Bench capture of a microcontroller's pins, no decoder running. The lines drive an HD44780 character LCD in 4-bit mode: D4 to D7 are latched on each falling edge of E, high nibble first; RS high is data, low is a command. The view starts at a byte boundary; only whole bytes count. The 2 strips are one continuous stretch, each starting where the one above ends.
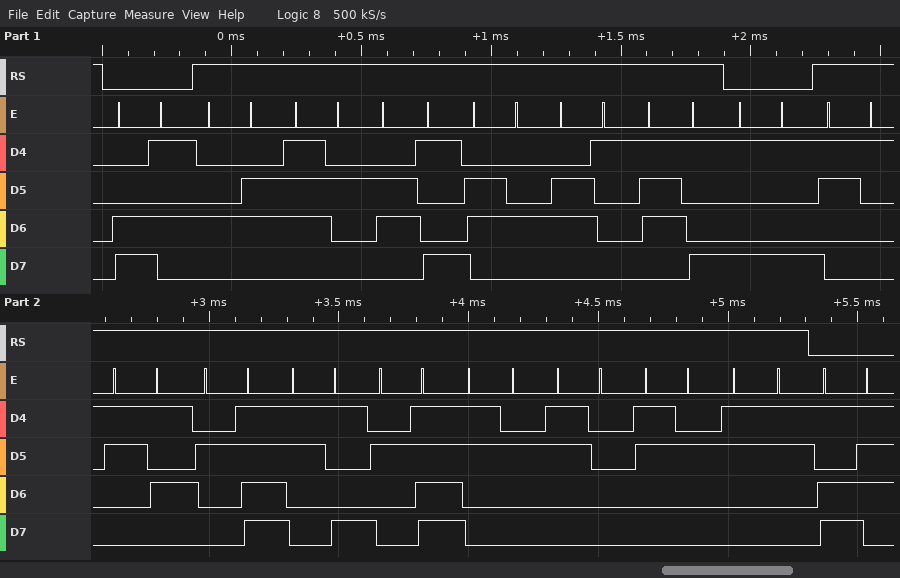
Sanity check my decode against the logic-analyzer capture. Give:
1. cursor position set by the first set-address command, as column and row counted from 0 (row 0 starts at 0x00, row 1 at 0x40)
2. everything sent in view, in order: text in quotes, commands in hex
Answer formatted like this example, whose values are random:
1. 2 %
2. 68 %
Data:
1. column 5, row 1
2. 0xC5 "Friday" 0x99 "15/9/2023" 0xD7
